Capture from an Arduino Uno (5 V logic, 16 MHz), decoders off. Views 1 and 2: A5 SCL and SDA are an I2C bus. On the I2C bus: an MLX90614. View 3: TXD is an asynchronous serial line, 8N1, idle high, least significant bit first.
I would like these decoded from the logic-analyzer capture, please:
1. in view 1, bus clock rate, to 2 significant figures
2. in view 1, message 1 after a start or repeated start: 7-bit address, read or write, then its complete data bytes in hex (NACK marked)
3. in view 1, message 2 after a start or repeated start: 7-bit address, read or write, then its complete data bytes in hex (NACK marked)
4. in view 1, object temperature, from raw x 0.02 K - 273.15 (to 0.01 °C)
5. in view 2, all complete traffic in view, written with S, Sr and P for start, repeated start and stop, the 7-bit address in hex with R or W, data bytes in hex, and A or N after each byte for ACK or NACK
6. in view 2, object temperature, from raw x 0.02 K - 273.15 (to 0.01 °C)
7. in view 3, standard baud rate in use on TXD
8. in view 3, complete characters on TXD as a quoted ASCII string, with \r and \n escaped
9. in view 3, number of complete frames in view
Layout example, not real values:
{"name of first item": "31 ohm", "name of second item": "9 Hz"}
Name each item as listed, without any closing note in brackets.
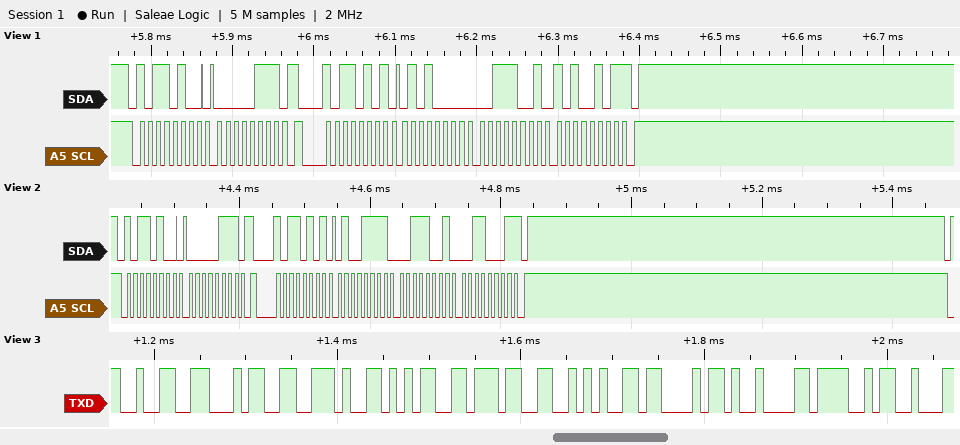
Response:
{"in view 1, bus clock rate, to 2 significant figures": "100 kHz", "in view 1, message 1 after a start or repeated start: 7-bit address, read or write, then its complete data bytes in hex": "0x5A write: 07", "in view 1, message 2 after a start or repeated start: 7-bit address, read or write, then its complete data bytes in hex": "0x5A read: 50 39 A5 NACK", "in view 1, object temperature, from raw x 0.02 K - 273.15": "20.29 °C", "in view 2, all complete traffic in view, written with S, Sr and P for start, repeated start and stop, the 7-bit address in hex with R or W, data bytes in hex, and A or N after each byte for ACK or NACK": "S 5AW A 07 A Sr 5AR A 4F A 39 A 31 N P", "in view 2, object temperature, from raw x 0.02 K - 273.15": "20.27 °C", "in view 3, standard baud rate in use on TXD": "115200 baud", "in view 3, complete characters on TXD as a quoted ASCII string, with \\r and \\n escaped": "\"24.57*C\\tO\"", "in view 3, number of complete frames in view": "9"}
